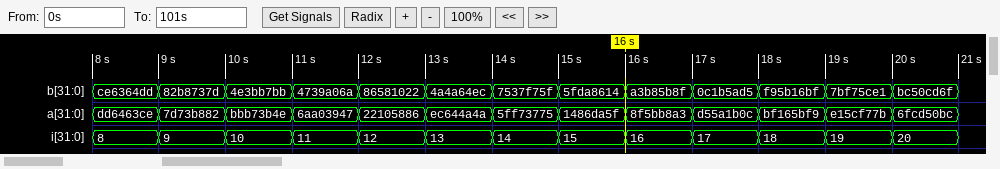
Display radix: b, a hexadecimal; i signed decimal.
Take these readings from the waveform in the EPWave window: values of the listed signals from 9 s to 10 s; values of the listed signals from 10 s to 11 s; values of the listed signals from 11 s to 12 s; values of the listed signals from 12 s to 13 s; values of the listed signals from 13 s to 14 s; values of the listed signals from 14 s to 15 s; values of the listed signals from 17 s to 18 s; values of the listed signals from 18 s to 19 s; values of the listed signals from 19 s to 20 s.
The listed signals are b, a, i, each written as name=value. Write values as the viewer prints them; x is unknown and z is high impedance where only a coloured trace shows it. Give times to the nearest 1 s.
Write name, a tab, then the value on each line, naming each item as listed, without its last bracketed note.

values of the listed signals from 9 s to 10 s	b=82b8737d, a=7d73b882, i=9
values of the listed signals from 10 s to 11 s	b=4e3bb7bb, a=bbb73b4e, i=10
values of the listed signals from 11 s to 12 s	b=4739a06a, a=6aa03947, i=11
values of the listed signals from 12 s to 13 s	b=86581022, a=22105886, i=12
values of the listed signals from 13 s to 14 s	b=4a4a64ec, a=ec644a4a, i=13
values of the listed signals from 14 s to 15 s	b=7537f75f, a=5ff73775, i=14
values of the listed signals from 17 s to 18 s	b=0c1b5ad5, a=d55a1b0c, i=17
values of the listed signals from 18 s to 19 s	b=f95b16bf, a=bf165bf9, i=18
values of the listed signals from 19 s to 20 s	b=7bf75ce1, a=e15cf77b, i=19
